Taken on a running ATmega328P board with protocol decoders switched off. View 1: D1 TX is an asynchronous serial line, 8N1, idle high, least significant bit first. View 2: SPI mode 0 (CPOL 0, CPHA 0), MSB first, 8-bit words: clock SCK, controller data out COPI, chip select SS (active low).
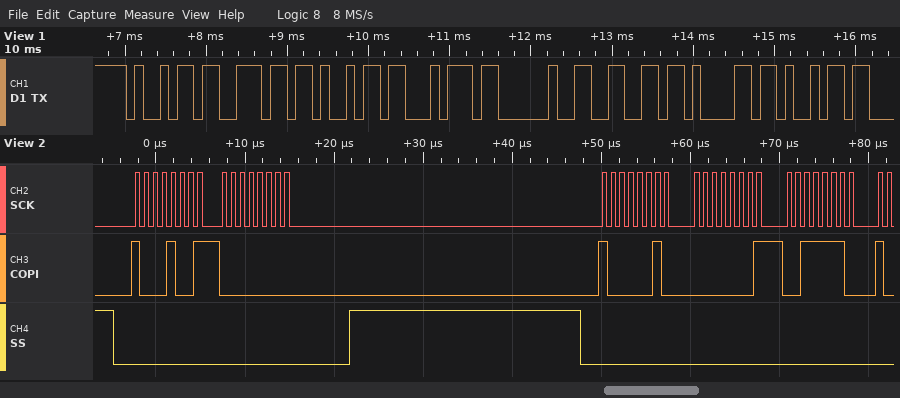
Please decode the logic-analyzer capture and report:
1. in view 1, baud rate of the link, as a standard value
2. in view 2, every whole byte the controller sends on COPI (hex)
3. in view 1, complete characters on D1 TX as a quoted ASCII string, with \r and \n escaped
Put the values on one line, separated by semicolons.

9600 baud; 0x89 0x00 0x82 0x01 0x3E; "init fai"
